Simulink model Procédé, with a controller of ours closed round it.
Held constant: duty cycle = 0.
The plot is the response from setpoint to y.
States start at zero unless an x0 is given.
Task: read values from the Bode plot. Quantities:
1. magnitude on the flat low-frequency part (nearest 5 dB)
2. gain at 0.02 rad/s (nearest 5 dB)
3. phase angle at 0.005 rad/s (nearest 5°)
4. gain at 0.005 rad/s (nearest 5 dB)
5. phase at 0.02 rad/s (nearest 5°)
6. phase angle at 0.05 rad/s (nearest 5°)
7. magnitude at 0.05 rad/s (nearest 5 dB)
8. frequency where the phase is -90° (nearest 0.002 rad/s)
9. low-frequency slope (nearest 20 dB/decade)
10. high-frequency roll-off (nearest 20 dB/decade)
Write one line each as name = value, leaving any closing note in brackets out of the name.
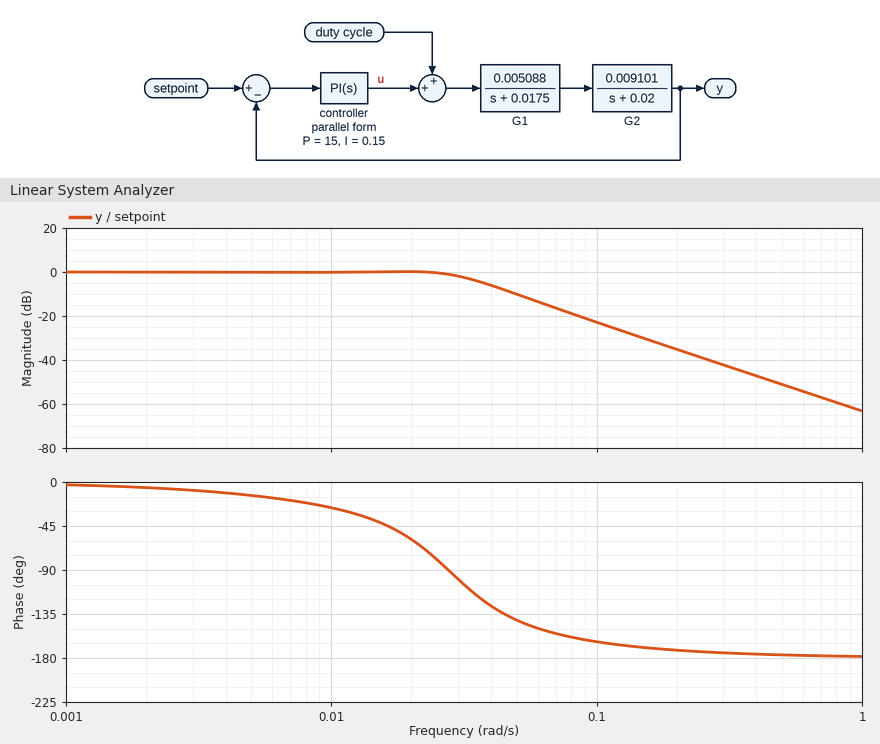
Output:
magnitude on the flat low-frequency part = 0 dB
gain at 0.02 rad/s = 0 dB
phase angle at 0.005 rad/s = -15°
gain at 0.005 rad/s = 0 dB
phase at 0.02 rad/s = -60°
phase angle at 0.05 rad/s = -140°
magnitude at 0.05 rad/s = -10 dB
frequency where the phase is -90° = 0.028 rad/s
low-frequency slope = 0 dB/decade
high-frequency roll-off = -40 dB/decade
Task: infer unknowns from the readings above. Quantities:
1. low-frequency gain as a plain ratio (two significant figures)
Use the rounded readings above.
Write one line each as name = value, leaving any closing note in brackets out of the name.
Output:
low-frequency gain as a plain ratio = 1.0
